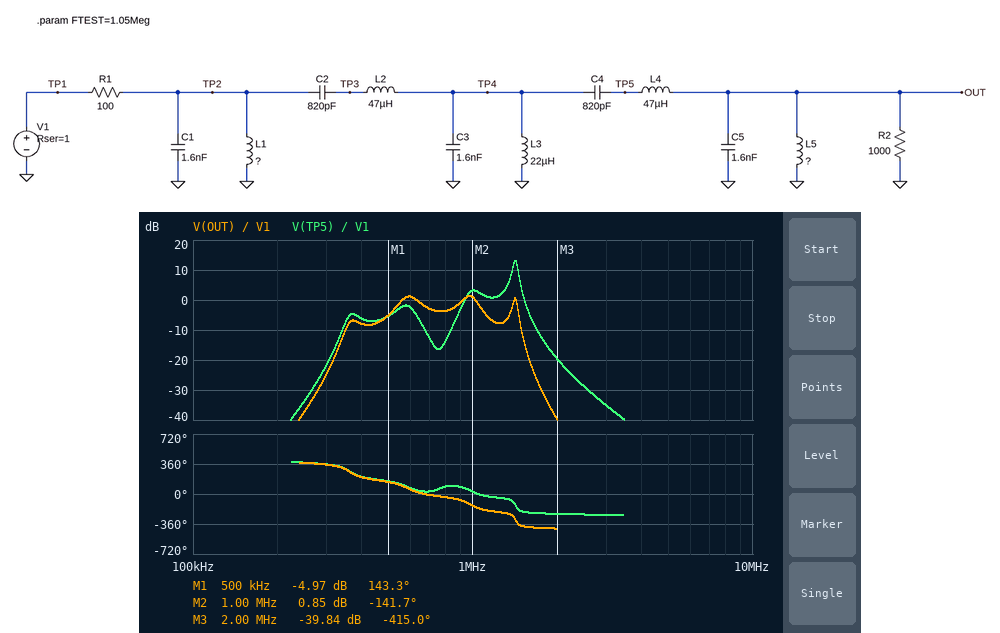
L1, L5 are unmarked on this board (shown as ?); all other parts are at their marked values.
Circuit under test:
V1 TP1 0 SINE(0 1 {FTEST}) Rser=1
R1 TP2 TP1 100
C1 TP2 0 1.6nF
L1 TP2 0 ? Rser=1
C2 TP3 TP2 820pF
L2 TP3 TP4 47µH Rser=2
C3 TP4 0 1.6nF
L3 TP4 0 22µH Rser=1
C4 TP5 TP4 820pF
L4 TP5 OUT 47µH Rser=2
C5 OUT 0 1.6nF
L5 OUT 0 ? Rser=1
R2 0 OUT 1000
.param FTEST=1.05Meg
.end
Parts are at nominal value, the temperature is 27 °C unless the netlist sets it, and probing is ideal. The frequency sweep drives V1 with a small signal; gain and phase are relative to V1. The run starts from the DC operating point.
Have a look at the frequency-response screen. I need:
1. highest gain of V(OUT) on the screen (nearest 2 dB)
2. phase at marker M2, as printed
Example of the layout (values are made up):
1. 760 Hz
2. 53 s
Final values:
1. 2 dB
2. -141.7 deg
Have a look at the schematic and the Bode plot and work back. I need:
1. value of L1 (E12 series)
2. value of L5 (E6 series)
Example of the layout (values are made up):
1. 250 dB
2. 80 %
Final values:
1. 68 µH
2. 68 µH
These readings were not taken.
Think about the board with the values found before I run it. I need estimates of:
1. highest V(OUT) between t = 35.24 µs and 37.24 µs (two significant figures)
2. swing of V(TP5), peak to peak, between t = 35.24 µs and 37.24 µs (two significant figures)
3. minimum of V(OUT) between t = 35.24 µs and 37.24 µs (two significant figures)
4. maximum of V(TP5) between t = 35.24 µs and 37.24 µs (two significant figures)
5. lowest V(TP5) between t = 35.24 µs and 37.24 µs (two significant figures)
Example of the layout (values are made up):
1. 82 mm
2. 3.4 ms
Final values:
1. 830 mV
2. 2.7 V
3. -830 mV
4. 1.3 V
5. -1.3 V
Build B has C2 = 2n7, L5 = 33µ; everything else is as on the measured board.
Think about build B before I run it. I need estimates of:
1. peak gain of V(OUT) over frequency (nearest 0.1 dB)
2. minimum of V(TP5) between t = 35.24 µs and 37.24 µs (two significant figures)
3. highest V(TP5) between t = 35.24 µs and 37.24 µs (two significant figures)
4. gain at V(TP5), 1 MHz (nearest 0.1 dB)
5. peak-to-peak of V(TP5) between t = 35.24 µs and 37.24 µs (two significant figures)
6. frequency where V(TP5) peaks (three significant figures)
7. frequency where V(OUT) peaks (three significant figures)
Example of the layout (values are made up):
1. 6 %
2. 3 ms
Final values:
1. 3.2 dB
2. -530 mV
3. 530 mV
4. -6.0 dB
5. 1.1 V
6. 1.39 MHz
7. 904 kHz
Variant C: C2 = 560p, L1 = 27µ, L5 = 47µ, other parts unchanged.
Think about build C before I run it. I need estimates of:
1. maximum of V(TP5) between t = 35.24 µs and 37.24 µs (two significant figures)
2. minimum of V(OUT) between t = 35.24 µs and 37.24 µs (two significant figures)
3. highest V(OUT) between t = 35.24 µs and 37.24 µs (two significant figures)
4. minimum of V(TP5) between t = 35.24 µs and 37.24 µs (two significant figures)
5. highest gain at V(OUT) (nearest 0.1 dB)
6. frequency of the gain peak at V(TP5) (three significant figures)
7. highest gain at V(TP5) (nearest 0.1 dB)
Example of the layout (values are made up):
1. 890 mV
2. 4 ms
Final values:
1. 1.5 V
2. -1.1 V
3. 1.1 V
4. -1.5 V
5. 2.7 dB
6. 1.46 MHz
7. 11.4 dB
